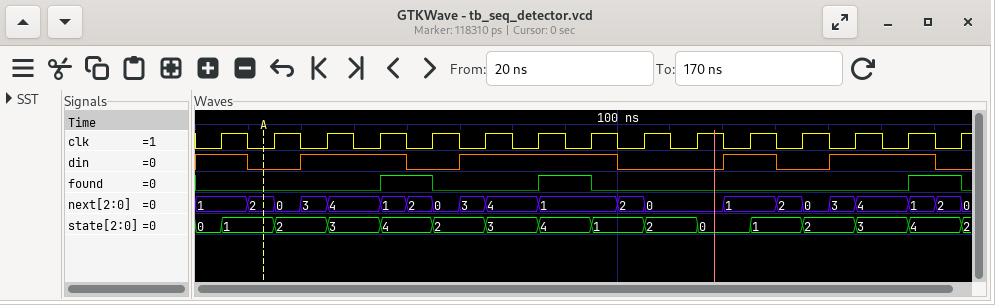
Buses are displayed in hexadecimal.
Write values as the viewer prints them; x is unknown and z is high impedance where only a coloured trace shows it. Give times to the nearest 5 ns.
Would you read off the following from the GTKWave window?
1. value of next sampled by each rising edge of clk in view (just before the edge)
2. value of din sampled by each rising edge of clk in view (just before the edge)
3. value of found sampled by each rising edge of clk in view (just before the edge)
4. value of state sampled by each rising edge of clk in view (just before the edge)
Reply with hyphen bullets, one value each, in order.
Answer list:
- 1, 2, 3, 4, 2, 3, 4, 1, 2, 0, 1, 2, 3, 4, 2
- 1 0 1 1 0 1 1 1 0 0 1 0 1 1 0
- 0 0 0 0 1 0 0 1 0 0 0 0 0 0 1
- 0, 1, 2, 3, 4, 2, 3, 4, 1, 2, 0, 1, 2, 3, 4
